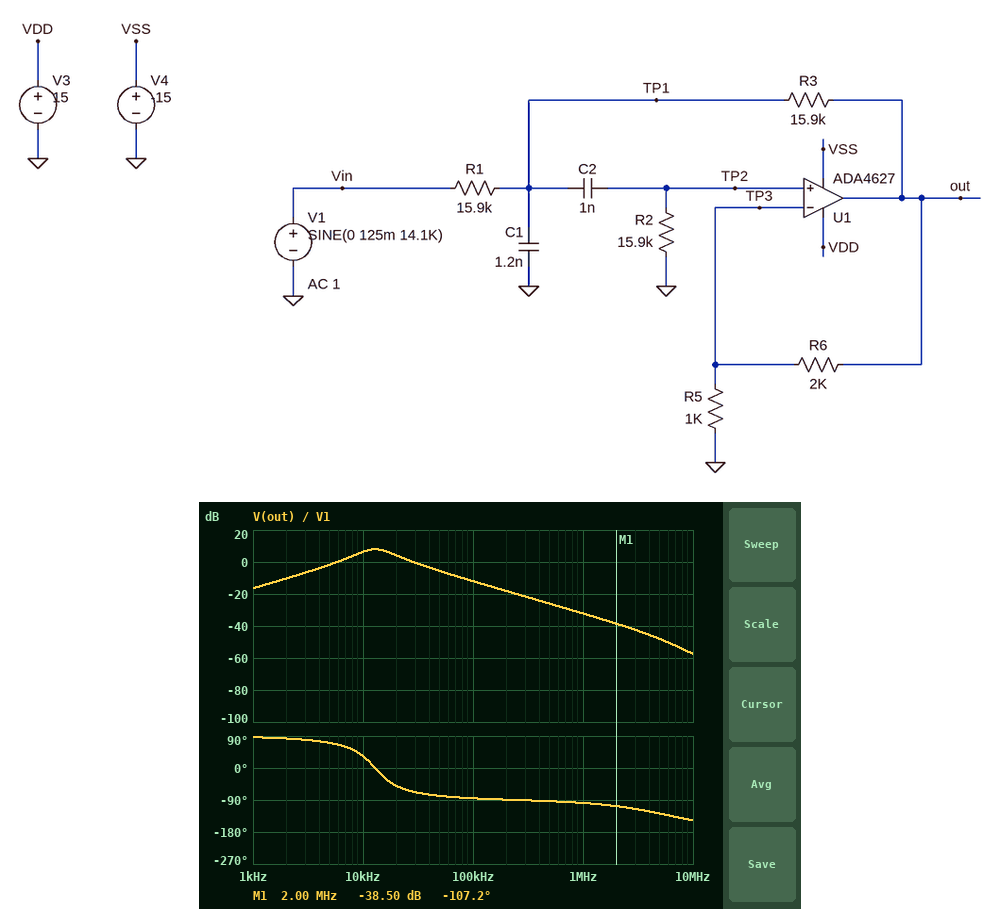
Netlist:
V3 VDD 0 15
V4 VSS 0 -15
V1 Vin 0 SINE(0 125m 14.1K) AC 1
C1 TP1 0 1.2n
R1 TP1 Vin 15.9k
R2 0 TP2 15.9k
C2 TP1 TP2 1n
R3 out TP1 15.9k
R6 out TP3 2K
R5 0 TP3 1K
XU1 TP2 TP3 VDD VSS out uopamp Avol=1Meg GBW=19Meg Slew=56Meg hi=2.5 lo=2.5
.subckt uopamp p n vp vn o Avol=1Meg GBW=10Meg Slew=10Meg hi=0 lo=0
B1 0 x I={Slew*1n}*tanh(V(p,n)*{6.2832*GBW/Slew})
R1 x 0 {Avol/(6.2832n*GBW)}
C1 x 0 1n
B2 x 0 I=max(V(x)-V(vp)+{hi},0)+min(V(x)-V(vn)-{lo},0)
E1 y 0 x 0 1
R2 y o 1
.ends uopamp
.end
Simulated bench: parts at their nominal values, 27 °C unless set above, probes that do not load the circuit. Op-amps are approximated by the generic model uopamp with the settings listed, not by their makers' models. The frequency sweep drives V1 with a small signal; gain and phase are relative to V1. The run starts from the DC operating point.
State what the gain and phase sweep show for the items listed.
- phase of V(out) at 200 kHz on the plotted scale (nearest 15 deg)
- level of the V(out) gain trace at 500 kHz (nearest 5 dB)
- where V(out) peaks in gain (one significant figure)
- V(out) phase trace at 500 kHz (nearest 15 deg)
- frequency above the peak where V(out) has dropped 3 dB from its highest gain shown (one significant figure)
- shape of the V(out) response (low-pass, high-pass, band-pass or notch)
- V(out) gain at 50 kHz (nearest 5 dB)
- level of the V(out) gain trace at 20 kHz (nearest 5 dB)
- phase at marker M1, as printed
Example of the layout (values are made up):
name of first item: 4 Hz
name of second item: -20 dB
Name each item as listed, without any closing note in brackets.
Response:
phase of V(out) at 200 kHz on the plotted scale: -90 deg
level of the V(out) gain trace at 500 kHz: -25 dB
where V(out) peaks in gain: 10 kHz
V(out) phase trace at 500 kHz: -90 deg
frequency above the peak where V(out) has dropped 3 dB from its highest gain shown: 20 kHz
shape of the V(out) response: band-pass
V(out) gain at 50 kHz: -5 dB
level of the V(out) gain trace at 20 kHz: 5 dB
phase at marker M1, as printed: -107.2 deg
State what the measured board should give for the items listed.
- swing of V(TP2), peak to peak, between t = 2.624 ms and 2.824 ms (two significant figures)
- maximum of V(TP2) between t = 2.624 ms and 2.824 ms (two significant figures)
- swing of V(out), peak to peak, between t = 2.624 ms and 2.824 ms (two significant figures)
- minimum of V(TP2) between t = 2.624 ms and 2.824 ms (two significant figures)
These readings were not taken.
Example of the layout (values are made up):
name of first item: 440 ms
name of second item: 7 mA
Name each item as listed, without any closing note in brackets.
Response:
swing of V(TP2), peak to peak, between t = 2.624 ms and 2.824 ms: 200 mV
maximum of V(TP2) between t = 2.624 ms and 2.824 ms: 100 mV
swing of V(out), peak to peak, between t = 2.624 ms and 2.824 ms: 610 mV
minimum of V(TP2) between t = 2.624 ms and 2.824 ms: -100 mV
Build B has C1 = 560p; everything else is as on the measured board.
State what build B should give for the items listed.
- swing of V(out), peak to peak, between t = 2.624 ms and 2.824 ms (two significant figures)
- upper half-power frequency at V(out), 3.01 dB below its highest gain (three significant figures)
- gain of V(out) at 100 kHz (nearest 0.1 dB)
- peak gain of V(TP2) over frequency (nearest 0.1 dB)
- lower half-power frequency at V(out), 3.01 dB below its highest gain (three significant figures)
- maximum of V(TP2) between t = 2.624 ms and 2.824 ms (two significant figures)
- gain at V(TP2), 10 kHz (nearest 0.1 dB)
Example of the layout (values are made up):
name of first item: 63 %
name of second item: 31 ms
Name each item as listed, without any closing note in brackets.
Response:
swing of V(out), peak to peak, between t = 2.624 ms and 2.824 ms: 890 mV
upper half-power frequency at V(out), 3.01 dB below its highest gain: 24.4 kHz
gain of V(out) at 100 kHz: -5.2 dB
peak gain of V(TP2) over frequency: 5.0 dB
lower half-power frequency at V(out), 3.01 dB below its highest gain: 14.5 kHz
maximum of V(TP2) between t = 2.624 ms and 2.824 ms: 150 mV
gain at V(TP2), 10 kHz: -3.8 dB
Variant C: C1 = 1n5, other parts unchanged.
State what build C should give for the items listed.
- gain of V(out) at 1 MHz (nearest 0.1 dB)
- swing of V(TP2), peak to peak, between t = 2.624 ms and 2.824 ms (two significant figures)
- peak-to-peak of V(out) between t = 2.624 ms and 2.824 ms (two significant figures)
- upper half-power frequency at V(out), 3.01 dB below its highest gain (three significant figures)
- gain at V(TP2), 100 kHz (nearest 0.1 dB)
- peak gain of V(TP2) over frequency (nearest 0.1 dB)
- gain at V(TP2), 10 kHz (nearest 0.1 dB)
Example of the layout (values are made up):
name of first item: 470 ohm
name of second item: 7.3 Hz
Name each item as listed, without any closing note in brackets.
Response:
gain of V(out) at 1 MHz: -34.1 dB
swing of V(TP2), peak to peak, between t = 2.624 ms and 2.824 ms: 150 mV
peak-to-peak of V(out) between t = 2.624 ms and 2.824 ms: 450 mV
upper half-power frequency at V(out), 3.01 dB below its highest gain: 17.6 kHz
gain at V(TP2), 100 kHz: -23.5 dB
peak gain of V(TP2) over frequency: -3.5 dB
gain at V(TP2), 10 kHz: -4.0 dB
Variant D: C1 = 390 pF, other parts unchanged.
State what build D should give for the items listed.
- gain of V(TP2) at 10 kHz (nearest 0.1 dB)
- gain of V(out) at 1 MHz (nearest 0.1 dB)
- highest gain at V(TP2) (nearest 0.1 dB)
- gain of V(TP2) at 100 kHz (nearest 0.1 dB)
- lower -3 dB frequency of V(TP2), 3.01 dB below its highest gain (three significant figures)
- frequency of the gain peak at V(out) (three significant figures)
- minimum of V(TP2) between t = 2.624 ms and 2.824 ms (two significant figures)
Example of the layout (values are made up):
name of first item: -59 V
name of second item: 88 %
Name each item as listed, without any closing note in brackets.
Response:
gain of V(TP2) at 10 kHz: -4.4 dB
gain of V(out) at 1 MHz: -22.5 dB
highest gain at V(TP2): 8.2 dB
gain of V(TP2) at 100 kHz: -11.5 dB
lower -3 dB frequency of V(TP2), 3.01 dB below its highest gain: 18.1 kHz
frequency of the gain peak at V(out): 22.5 kHz
minimum of V(TP2) between t = 2.624 ms and 2.824 ms: -130 mV
